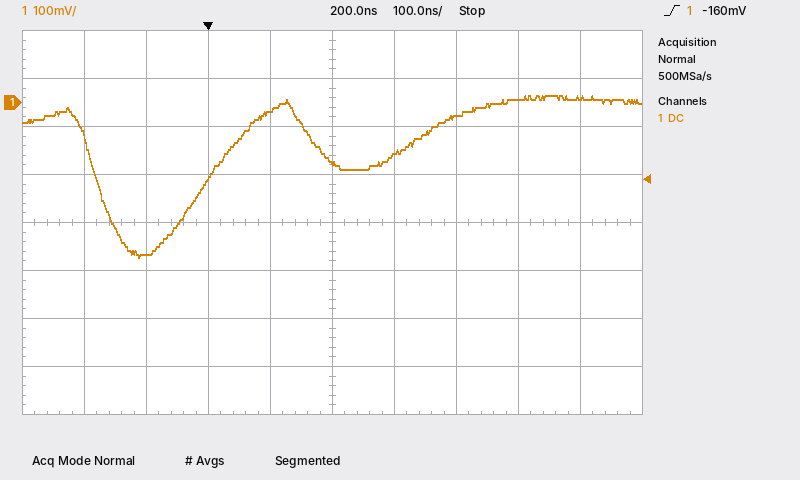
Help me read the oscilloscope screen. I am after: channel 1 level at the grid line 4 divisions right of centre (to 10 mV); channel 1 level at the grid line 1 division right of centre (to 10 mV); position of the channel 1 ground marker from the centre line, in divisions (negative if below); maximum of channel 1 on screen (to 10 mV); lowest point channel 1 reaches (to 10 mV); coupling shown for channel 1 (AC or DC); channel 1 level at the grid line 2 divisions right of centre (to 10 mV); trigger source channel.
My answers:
10 mV
-110 mV
+2.5 div
10 mV
-320 mV
DC
-30 mV
channel 1
